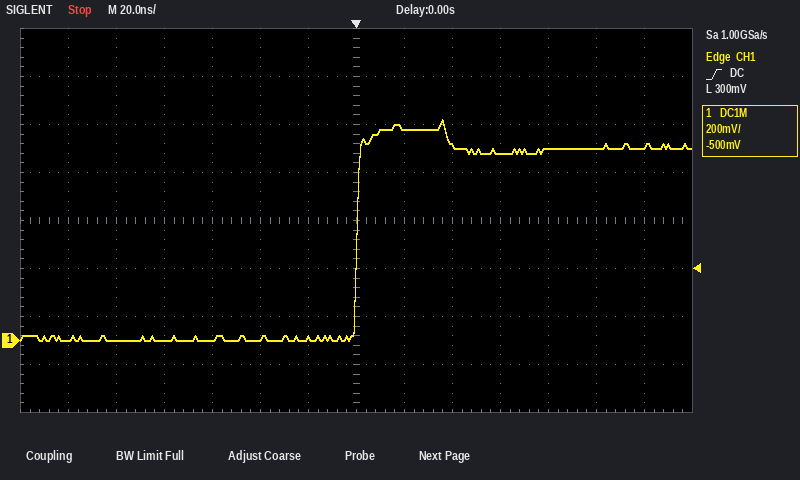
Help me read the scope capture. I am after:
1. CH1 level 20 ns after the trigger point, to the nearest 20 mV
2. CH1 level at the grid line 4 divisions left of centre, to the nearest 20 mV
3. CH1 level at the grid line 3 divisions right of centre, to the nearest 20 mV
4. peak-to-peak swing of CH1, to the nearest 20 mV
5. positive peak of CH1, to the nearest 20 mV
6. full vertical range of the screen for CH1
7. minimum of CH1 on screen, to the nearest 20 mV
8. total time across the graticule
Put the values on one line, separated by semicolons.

880 mV; 0 mV; 780 mV; 920 mV; 920 mV; 1.6 V; 0 mV; 280 ns
